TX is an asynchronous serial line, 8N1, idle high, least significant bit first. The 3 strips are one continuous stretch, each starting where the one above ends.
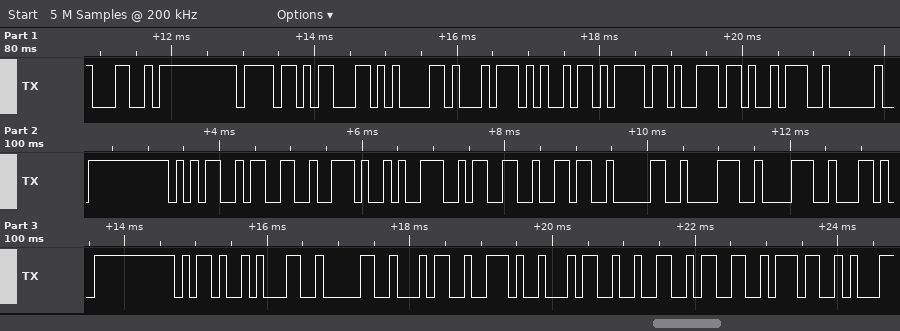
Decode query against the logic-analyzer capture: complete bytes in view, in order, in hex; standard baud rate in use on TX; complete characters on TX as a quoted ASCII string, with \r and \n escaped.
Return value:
4C 6F 63 61 74 69 6F 6E 3A 20 35 33 2E 39 33 36 30 38 38 2C 2D 31 30 34 2E 34 32 33 37
9600 baud
"Location: 53.936088,-104.4237"
